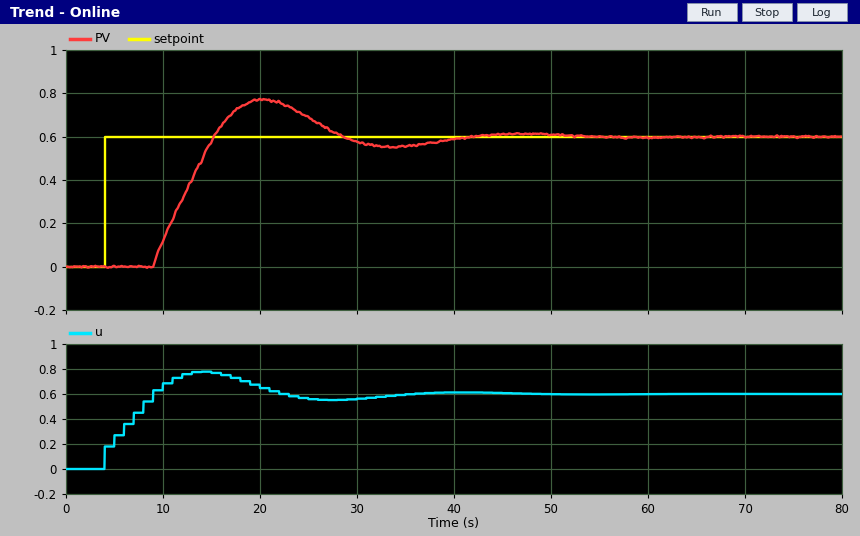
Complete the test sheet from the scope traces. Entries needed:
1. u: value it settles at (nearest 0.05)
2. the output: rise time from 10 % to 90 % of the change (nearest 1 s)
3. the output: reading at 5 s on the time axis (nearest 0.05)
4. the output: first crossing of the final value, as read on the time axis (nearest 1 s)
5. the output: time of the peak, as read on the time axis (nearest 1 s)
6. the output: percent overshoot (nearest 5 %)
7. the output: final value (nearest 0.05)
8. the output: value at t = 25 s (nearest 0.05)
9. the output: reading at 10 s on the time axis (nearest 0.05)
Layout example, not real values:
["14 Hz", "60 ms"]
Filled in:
["0.60", "5 s", "0.00", "15 s", "20 s", "30 %", "0.60", "0.70", "0.10"]
